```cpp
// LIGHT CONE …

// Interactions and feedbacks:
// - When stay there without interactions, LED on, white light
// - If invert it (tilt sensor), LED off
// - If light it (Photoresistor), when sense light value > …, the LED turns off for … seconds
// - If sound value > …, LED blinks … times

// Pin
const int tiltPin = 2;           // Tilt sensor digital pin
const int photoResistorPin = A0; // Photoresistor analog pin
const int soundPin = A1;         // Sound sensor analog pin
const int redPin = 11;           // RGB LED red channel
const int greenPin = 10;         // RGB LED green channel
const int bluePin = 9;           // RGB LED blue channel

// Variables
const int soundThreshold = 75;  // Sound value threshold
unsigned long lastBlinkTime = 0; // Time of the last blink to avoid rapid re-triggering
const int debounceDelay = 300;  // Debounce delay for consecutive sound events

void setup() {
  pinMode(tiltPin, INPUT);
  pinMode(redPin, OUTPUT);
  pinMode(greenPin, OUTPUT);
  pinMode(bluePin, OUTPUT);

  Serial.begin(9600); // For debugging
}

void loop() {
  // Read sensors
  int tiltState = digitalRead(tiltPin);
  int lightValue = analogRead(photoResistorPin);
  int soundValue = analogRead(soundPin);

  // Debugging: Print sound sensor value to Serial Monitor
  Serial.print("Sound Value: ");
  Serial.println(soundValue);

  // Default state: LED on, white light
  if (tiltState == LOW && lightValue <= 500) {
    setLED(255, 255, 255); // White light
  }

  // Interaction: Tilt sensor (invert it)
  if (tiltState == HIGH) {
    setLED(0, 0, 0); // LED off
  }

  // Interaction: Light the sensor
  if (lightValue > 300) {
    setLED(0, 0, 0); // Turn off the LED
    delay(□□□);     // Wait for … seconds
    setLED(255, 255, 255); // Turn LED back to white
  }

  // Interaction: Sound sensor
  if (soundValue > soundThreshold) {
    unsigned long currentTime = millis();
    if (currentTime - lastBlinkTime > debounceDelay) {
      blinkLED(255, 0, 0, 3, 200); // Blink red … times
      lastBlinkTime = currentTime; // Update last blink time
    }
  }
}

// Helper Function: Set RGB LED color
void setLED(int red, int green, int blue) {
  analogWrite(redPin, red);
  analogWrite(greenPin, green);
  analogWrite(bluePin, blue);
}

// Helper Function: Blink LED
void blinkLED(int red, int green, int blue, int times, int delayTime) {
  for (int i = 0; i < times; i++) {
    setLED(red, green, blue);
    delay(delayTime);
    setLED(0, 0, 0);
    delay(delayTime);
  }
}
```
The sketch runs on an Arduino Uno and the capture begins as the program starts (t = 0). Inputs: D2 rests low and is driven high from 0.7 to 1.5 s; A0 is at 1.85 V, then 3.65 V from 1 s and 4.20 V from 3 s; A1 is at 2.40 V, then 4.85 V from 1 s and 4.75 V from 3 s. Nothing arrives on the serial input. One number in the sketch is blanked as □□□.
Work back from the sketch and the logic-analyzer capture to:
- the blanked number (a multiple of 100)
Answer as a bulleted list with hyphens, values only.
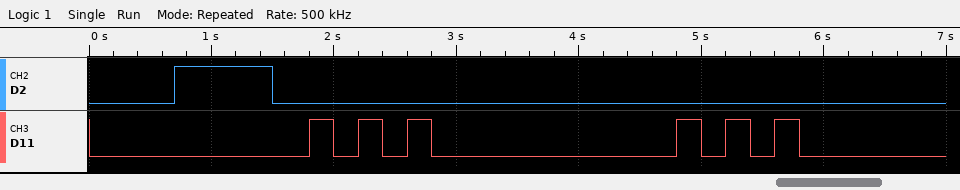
- 1800
